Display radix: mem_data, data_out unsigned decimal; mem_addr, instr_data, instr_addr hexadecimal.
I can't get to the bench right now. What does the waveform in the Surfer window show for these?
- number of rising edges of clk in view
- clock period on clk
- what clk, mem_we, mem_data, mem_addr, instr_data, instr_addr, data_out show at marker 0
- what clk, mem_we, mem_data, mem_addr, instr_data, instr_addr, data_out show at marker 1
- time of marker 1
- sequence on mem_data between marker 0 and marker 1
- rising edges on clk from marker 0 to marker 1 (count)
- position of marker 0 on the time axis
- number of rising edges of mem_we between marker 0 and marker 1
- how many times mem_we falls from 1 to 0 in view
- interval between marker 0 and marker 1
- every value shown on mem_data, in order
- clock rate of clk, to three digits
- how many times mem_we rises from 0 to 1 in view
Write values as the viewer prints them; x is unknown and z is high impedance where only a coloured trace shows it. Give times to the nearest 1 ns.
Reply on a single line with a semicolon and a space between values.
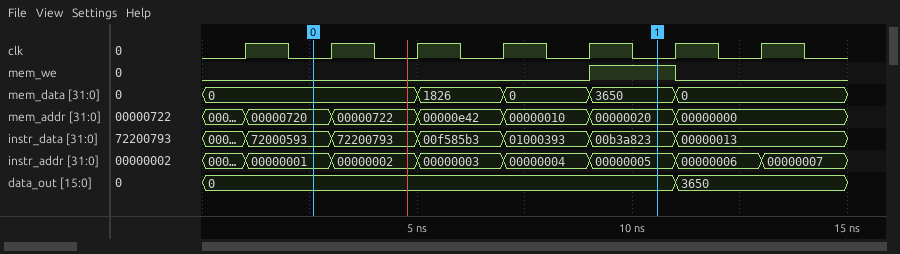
7; 2 ns; clk=0, mem_we=0, mem_data=0, mem_addr=00000720, instr_data=72000593, instr_addr=00000001, data_out=0; clk=0, mem_we=1, mem_data=3650, mem_addr=00000020, instr_data=00b3a823, instr_addr=00000005, data_out=0; 11 ns; 0, 1826, 0, 3650; 4; 3 ns; 1; 1; 8 ns; 0, 1826, 0, 3650, 0; 500 MHz; 1
